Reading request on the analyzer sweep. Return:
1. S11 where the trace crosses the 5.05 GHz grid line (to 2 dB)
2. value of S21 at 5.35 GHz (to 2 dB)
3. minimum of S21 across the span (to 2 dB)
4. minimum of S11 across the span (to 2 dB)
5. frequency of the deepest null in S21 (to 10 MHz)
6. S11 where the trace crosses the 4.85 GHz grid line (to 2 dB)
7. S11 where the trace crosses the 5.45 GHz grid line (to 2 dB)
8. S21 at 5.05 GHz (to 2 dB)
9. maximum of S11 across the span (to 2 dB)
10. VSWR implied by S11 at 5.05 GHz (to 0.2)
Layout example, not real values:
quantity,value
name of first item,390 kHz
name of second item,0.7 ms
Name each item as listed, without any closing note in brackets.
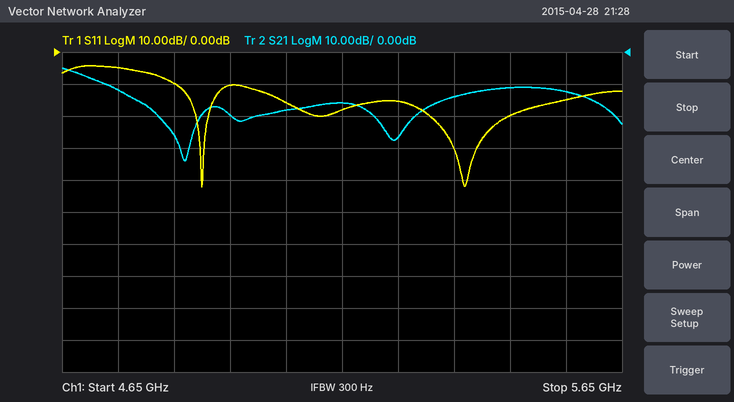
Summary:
quantity,value
S11 where the trace crosses the 5.05 GHz grid line,-16 dB
value of S21 at 5.35 GHz,-14 dB
minimum of S21 across the span,-34 dB
minimum of S11 across the span,-42 dB
frequency of the deepest null in S21,4.87 GHz
S11 where the trace crosses the 4.85 GHz grid line,-10 dB
S11 where the trace crosses the 5.45 GHz grid line,-20 dB
S21 at 5.05 GHz,-18 dB
maximum of S11 across the span,-4 dB
VSWR implied by S11 at 5.05 GHz,1.4
